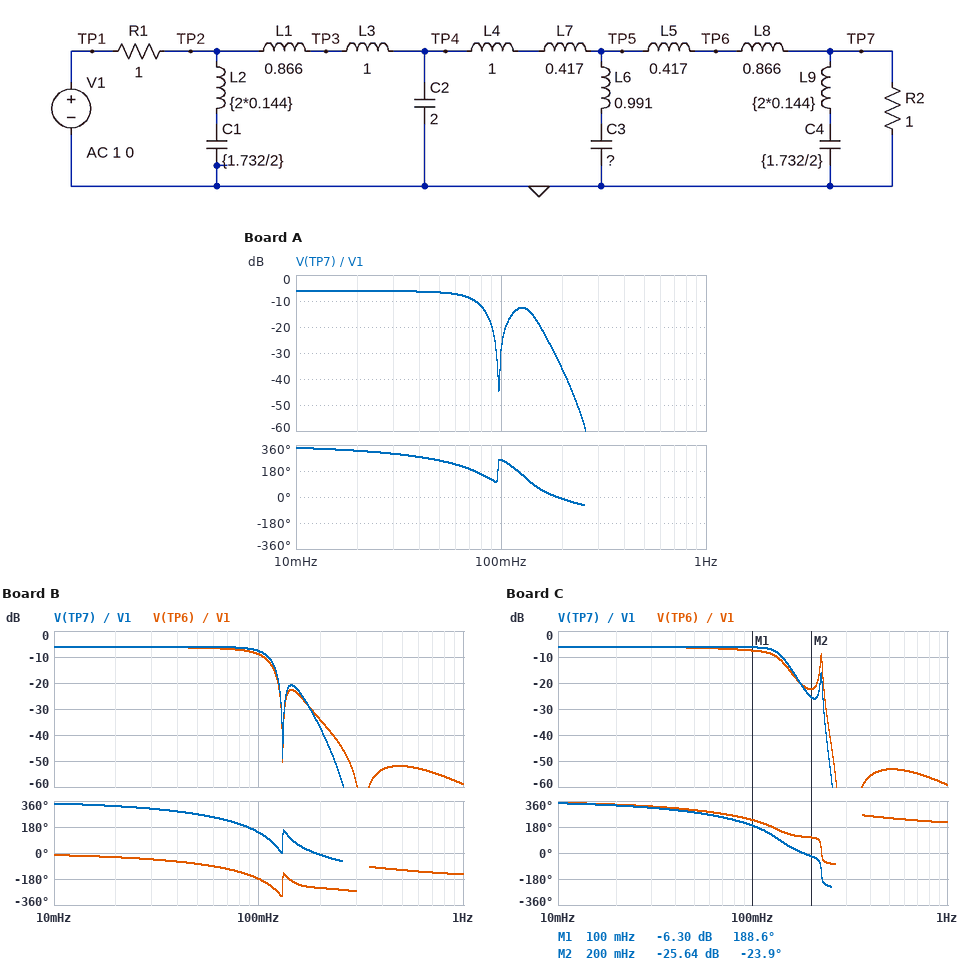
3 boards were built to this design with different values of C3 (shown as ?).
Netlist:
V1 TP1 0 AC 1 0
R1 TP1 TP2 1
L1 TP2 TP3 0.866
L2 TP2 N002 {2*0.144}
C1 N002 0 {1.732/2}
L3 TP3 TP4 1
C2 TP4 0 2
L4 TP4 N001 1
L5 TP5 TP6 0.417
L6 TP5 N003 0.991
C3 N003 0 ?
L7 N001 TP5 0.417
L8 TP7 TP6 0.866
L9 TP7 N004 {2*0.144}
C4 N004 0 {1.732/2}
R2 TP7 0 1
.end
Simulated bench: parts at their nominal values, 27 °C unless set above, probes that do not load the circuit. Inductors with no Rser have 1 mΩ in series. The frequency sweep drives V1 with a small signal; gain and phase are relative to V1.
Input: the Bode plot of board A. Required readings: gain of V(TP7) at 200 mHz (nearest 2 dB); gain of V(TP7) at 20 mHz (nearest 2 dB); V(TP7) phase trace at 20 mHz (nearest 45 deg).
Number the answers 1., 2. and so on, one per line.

1. -36 dB
2. -6 dB
3. 315 deg
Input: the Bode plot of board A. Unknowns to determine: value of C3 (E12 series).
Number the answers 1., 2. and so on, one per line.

1. 2.7 F
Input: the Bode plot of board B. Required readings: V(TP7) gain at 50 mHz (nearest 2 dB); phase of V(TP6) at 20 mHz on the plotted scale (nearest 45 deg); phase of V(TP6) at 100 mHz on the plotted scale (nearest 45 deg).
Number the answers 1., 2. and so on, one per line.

1. -6 dB
2. -45 deg
3. -180 deg
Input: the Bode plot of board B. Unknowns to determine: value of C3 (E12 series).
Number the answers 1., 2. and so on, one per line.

1. 1.5 F
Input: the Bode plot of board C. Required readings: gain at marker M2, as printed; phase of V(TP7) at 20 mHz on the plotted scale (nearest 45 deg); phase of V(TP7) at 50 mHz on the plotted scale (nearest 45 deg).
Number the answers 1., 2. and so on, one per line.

1. -25.64 dB
2. 315 deg
3. 270 deg
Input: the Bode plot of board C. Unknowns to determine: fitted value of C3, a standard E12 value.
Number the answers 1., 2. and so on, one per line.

1. 330 mF
